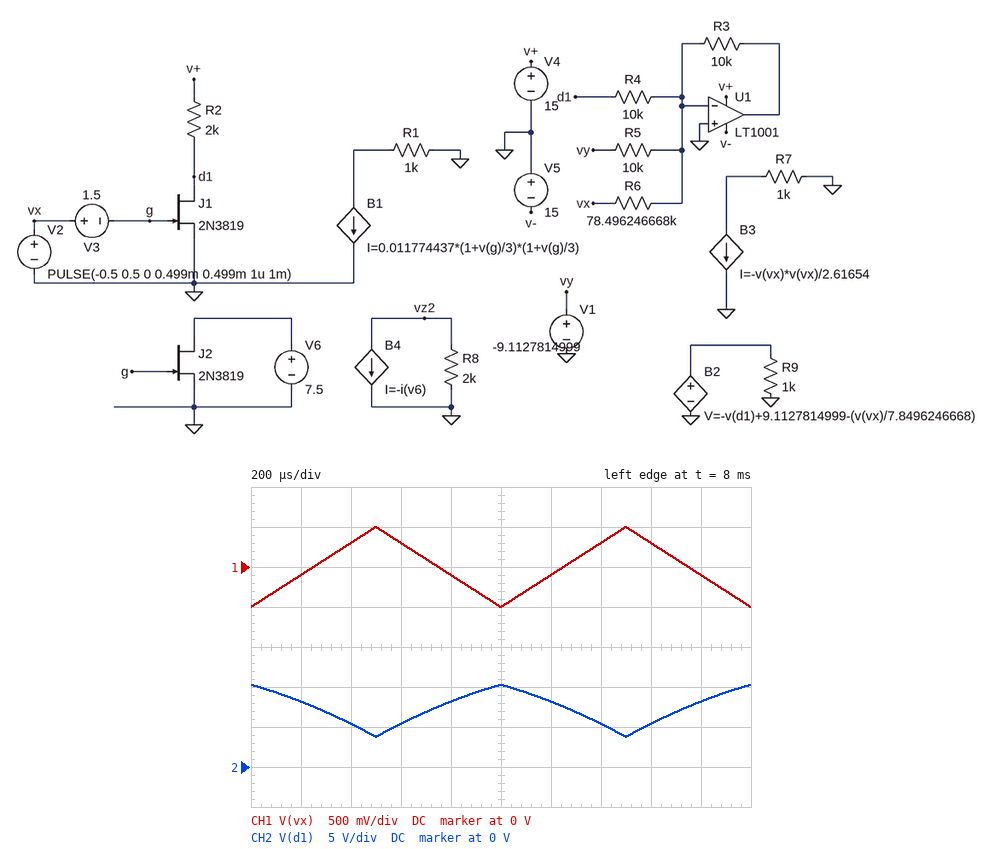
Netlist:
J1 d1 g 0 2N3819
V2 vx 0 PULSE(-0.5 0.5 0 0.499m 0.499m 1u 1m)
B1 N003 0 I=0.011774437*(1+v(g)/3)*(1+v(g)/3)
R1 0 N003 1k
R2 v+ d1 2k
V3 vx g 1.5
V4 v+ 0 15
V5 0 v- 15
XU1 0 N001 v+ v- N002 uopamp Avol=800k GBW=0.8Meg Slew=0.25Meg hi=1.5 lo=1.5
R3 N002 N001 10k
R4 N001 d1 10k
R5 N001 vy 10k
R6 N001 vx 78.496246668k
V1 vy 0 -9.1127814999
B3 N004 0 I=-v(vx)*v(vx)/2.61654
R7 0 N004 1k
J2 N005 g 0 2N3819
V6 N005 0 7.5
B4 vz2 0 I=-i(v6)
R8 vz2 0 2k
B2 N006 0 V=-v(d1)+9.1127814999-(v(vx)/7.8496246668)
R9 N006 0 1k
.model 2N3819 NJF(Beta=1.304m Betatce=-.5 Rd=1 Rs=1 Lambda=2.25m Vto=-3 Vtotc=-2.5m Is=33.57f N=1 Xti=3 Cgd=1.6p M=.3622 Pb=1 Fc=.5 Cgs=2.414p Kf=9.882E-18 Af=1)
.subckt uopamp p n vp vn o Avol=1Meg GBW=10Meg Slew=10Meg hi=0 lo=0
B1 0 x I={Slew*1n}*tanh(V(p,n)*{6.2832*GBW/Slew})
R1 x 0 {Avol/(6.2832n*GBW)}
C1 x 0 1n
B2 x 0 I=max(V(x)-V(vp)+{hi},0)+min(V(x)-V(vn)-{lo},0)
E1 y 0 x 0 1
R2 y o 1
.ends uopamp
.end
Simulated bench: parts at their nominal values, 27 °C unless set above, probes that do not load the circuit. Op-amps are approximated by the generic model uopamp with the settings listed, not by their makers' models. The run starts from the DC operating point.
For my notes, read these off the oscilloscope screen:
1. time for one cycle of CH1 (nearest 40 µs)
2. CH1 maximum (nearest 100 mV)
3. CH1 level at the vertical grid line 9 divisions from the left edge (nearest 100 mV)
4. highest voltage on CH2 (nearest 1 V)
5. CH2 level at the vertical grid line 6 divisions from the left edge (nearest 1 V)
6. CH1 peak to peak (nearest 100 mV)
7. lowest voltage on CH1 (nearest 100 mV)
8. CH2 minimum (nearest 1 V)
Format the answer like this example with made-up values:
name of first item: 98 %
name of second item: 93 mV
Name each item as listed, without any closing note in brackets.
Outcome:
time for one cycle of CH1: 1.00 ms
CH1 maximum: 500 mV
CH1 level at the vertical grid line 9 divisions from the left edge: -100 mV
highest voltage on CH2: 10 V
CH2 level at the vertical grid line 6 divisions from the left edge: 8 V
CH1 peak to peak: 1.0 V
lowest voltage on CH1: -500 mV
CH2 minimum: 4 V
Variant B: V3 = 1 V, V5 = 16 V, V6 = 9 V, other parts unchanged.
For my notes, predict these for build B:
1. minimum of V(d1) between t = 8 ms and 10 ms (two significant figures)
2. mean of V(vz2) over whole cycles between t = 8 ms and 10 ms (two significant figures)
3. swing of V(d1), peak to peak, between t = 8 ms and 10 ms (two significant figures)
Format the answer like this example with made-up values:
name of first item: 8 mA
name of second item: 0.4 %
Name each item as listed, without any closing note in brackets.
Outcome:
minimum of V(d1) between t = 8 ms and 10 ms: 1.4 V
mean of V(vz2) over whole cycles between t = 8 ms and 10 ms: -11 V
swing of V(d1), peak to peak, between t = 8 ms and 10 ms: 6.1 V
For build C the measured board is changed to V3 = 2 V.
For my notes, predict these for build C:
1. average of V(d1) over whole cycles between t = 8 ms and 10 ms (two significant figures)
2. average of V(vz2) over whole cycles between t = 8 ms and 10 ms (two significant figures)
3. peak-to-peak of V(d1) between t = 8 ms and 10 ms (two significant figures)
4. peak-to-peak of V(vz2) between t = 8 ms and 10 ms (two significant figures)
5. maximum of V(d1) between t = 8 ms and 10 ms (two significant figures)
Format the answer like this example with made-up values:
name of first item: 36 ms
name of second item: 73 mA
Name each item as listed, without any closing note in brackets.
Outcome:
average of V(d1) over whole cycles between t = 8 ms and 10 ms: 10 V
average of V(vz2) over whole cycles between t = 8 ms and 10 ms: -2.9 V
peak-to-peak of V(d1) between t = 8 ms and 10 ms: 4.4 V
peak-to-peak of V(vz2) between t = 8 ms and 10 ms: 5.3 V
maximum of V(d1) between t = 8 ms and 10 ms: 12 V
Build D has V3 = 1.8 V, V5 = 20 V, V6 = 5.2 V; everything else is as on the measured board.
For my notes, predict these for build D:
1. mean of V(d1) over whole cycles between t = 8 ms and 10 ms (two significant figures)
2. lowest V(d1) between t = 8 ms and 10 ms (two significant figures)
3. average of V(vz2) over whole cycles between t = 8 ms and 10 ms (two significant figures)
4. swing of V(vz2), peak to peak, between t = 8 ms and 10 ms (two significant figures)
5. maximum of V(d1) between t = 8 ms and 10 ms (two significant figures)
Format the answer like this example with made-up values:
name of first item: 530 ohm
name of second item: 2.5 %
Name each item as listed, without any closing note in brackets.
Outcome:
mean of V(d1) over whole cycles between t = 8 ms and 10 ms: 9.1 V
lowest V(d1) between t = 8 ms and 10 ms: 6.2 V
average of V(vz2) over whole cycles between t = 8 ms and 10 ms: -4.0 V
swing of V(vz2), peak to peak, between t = 8 ms and 10 ms: 6.3 V
maximum of V(d1) between t = 8 ms and 10 ms: 11 V
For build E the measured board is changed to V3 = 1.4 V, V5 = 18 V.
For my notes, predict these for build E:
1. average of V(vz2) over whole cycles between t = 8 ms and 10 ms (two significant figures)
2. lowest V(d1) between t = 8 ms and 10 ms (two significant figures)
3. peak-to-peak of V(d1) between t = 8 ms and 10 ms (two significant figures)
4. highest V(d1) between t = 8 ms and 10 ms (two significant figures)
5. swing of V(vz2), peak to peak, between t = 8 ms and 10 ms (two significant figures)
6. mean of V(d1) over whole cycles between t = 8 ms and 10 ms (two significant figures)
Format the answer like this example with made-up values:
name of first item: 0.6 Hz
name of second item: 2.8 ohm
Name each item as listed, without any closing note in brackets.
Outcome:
average of V(vz2) over whole cycles between t = 8 ms and 10 ms: -7.0 V
lowest V(d1) between t = 8 ms and 10 ms: 2.9 V
peak-to-peak of V(d1) between t = 8 ms and 10 ms: 6.9 V
highest V(d1) between t = 8 ms and 10 ms: 9.8 V
swing of V(vz2), peak to peak, between t = 8 ms and 10 ms: 8.4 V
mean of V(d1) over whole cycles between t = 8 ms and 10 ms: 6.7 V
